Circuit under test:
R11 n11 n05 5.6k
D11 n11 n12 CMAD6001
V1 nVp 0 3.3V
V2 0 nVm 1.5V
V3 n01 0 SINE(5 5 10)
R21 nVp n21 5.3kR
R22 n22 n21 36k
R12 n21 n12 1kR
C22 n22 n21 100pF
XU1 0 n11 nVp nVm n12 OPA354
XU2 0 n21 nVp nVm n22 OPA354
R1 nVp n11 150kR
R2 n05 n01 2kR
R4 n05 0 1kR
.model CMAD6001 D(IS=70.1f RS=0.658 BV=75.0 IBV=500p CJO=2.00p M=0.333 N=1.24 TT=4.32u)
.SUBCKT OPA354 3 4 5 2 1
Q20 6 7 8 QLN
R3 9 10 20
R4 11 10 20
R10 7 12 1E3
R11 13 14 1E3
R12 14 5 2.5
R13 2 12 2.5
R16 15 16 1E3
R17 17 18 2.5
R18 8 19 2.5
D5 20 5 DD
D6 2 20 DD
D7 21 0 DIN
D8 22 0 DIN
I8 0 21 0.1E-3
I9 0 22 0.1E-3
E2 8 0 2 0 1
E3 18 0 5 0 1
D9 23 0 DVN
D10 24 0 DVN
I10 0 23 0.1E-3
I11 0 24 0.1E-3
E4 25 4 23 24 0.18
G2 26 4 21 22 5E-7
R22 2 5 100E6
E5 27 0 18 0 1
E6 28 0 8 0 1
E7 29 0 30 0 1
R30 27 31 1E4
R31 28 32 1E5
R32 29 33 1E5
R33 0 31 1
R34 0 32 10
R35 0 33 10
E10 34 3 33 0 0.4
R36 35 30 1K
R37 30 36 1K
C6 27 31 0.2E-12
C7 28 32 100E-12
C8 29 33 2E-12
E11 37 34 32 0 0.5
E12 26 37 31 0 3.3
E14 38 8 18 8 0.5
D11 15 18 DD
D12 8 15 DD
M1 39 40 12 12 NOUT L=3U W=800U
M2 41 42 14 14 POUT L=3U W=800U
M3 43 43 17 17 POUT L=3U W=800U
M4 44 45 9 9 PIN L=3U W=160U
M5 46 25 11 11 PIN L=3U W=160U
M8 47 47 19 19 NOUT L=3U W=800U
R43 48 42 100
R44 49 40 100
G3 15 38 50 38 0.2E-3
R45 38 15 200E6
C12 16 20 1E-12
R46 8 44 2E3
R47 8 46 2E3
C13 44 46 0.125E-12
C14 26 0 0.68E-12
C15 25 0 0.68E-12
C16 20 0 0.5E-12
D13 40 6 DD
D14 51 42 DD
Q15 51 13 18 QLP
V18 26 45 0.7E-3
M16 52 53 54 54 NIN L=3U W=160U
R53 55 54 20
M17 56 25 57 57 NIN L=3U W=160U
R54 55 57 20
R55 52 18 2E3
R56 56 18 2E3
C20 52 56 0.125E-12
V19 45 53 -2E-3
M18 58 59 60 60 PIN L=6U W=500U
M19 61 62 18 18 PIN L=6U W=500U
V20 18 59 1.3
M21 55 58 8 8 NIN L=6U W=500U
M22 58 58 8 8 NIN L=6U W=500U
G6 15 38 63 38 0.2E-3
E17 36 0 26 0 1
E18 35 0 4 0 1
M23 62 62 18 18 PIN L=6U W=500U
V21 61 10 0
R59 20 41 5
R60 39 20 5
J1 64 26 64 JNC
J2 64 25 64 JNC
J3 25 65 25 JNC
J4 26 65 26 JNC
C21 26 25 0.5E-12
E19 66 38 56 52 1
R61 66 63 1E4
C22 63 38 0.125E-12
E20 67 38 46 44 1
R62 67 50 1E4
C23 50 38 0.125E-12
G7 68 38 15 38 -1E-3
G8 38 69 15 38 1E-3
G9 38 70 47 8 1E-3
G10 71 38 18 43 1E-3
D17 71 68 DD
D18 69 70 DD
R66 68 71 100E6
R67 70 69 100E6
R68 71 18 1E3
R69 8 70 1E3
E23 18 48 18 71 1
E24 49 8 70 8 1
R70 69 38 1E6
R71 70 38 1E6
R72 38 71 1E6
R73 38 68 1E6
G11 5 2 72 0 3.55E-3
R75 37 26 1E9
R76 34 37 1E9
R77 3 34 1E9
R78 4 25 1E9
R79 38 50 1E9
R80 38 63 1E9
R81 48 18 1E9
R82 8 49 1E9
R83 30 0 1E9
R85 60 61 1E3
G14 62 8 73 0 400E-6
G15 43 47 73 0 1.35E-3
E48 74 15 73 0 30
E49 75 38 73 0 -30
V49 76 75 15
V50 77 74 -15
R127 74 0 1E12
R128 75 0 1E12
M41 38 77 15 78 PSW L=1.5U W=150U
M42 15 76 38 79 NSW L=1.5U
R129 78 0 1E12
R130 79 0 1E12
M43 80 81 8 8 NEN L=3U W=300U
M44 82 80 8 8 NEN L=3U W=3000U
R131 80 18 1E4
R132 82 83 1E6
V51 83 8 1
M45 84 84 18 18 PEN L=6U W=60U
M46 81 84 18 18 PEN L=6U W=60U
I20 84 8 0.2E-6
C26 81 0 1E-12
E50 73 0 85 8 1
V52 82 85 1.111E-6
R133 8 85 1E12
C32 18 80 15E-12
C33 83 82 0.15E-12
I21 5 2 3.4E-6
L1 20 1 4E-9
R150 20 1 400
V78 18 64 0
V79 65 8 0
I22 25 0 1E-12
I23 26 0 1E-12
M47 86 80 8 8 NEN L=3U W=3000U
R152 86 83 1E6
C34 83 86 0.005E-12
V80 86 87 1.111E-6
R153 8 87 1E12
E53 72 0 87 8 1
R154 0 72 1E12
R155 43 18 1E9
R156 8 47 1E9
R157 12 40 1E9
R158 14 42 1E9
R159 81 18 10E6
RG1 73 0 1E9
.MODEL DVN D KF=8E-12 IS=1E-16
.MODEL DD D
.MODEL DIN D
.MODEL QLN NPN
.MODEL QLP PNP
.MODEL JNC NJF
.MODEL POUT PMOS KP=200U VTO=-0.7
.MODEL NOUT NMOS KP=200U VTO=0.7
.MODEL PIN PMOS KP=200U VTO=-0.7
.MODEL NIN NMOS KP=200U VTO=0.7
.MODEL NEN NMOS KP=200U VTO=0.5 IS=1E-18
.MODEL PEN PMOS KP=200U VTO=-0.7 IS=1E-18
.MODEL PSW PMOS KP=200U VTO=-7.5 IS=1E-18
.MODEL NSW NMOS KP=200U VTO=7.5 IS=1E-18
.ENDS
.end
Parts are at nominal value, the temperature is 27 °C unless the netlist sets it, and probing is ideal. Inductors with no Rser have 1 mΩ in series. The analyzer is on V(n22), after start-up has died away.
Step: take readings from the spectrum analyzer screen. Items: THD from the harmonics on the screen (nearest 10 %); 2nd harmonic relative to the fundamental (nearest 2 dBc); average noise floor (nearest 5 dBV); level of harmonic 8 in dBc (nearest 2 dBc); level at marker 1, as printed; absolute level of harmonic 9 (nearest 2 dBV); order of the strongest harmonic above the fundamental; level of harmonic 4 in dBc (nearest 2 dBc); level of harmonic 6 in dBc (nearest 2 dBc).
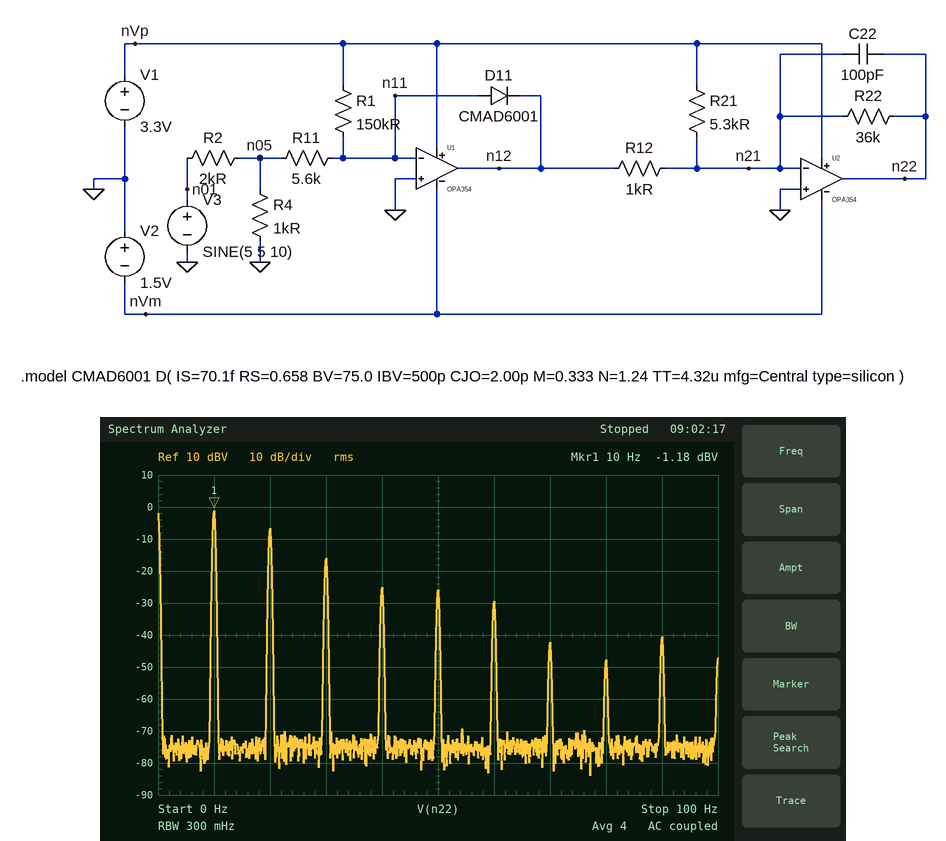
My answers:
60 %
-6 dBc
-75 dBV
-46 dBc
-1.18 dBV
-40 dBV
2
-24 dBc
-28 dBc
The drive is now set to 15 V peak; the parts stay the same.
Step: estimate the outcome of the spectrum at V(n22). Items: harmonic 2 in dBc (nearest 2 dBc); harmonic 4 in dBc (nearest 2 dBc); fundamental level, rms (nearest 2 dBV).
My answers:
-12 dBc
-14 dBc
6 dBV
